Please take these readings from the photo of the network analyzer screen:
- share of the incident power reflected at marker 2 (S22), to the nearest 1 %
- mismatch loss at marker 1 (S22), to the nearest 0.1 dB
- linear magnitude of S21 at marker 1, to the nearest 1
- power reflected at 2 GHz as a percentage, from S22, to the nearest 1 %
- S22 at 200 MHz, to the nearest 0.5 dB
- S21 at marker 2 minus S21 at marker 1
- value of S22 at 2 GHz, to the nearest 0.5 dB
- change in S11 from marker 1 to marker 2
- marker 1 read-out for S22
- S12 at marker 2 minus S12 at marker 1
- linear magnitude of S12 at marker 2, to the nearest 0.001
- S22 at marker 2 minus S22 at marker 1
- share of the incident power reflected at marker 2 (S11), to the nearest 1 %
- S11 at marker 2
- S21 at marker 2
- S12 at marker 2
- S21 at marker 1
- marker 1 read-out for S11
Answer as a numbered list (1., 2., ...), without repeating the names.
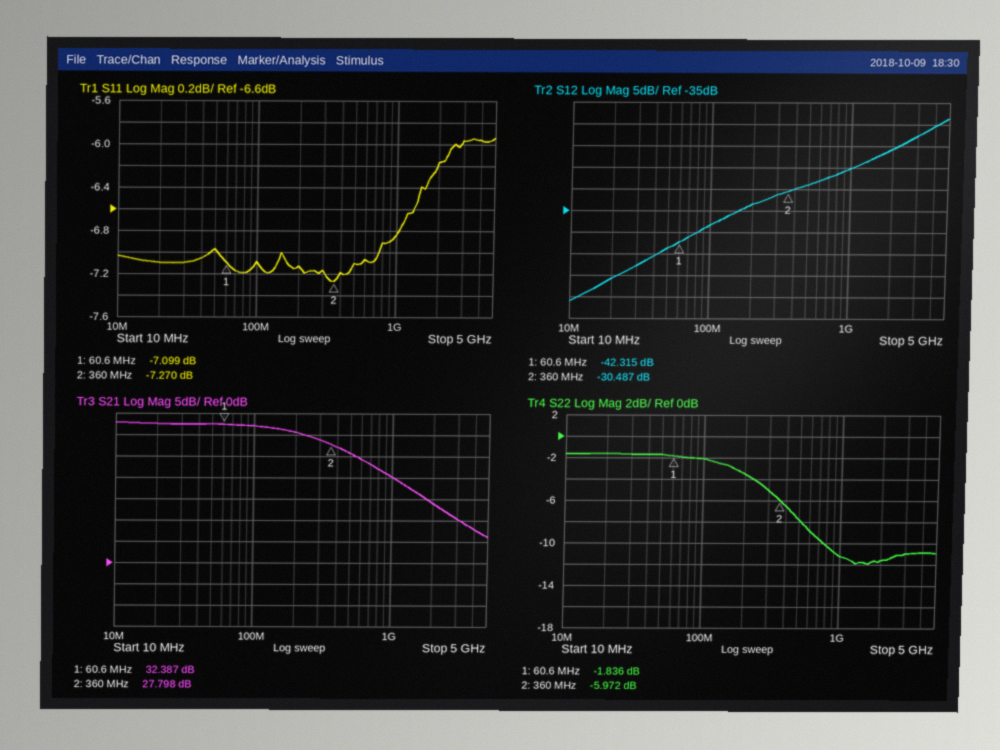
1. 25 %
2. 4.6 dB
3. 42
4. 7 %
5. -3.5 dB
6. -4.589 dB
7. -11.5 dB
8. -0.171 dB
9. -1.836 dB
10. 11.828 dB
11. 0.030
12. -4.136 dB
13. 19 %
14. -7.270 dB
15. 27.798 dB
16. -30.487 dB
17. 32.387 dB
18. -7.099 dB
